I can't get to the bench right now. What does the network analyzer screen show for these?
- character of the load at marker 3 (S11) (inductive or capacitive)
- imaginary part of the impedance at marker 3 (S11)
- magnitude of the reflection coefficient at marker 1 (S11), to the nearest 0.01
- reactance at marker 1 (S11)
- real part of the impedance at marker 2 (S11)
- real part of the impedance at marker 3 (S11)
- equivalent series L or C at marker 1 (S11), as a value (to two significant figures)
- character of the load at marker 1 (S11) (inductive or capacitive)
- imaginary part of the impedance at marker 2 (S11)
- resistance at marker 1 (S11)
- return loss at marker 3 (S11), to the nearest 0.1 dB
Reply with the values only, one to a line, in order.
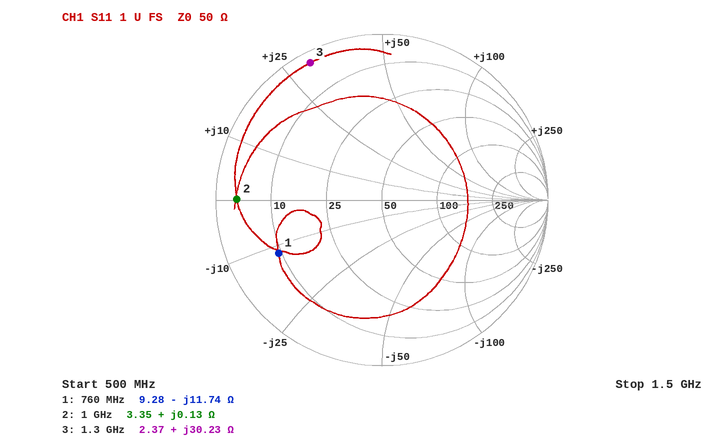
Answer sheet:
inductive
+30.23 Ω
0.70
-11.74 Ω
3.35 Ω
2.37 Ω
18 pF
capacitive
+0.13 Ω
9.28 Ω
0.6 dB
